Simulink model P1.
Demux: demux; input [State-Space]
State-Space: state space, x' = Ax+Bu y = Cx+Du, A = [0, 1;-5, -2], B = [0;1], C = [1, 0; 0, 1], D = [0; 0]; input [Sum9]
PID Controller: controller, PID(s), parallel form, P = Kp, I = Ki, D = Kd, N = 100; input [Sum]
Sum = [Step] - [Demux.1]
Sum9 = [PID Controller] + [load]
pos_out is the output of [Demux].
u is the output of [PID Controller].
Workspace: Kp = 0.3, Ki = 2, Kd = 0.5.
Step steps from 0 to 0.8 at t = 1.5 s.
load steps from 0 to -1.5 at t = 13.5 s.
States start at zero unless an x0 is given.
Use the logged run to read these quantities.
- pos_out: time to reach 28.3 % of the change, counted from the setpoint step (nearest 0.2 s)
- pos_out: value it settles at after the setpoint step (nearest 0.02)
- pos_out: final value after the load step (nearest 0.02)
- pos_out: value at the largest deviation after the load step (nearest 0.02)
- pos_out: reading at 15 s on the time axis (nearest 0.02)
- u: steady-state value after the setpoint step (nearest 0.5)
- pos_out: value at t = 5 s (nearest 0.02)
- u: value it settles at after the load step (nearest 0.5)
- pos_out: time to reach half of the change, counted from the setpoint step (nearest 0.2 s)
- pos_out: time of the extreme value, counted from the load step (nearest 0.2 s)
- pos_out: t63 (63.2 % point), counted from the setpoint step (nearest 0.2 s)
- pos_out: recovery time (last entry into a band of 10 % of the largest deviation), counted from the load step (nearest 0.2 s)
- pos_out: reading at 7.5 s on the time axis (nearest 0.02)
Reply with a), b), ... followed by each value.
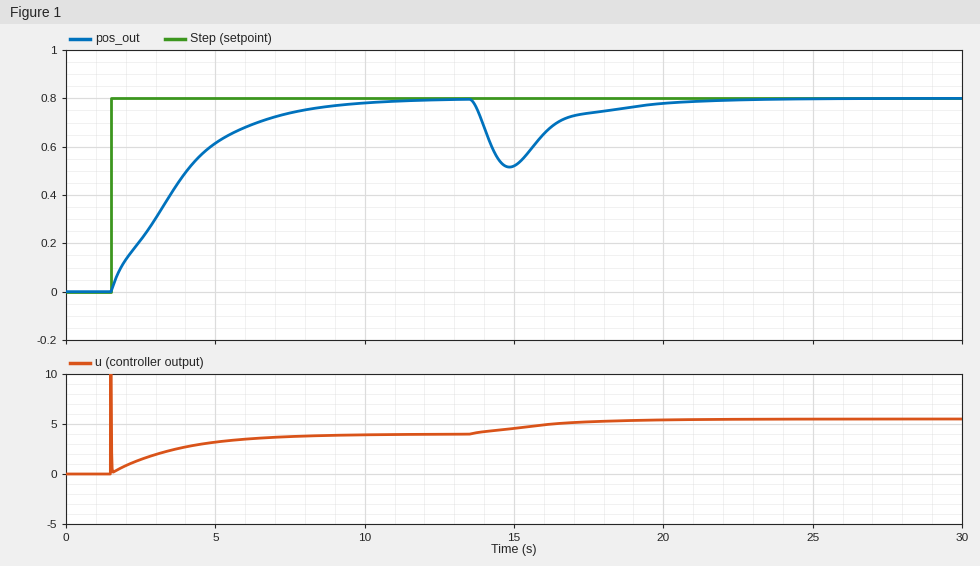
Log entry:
a) 1.0 s
b) 0.80
c) 0.80
d) 0.52
e) 0.52
f) 4.0
g) 0.62
h) 5.5
i) 2.0 s
j) 1.4 s
k) 2.6 s
l) 6.0 s
m) 0.74
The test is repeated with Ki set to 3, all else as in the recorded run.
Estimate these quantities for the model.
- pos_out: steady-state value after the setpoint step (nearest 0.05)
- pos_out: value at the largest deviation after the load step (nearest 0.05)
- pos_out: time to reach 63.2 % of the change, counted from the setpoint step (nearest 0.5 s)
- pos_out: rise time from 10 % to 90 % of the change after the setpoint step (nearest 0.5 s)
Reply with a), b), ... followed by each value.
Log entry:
a) 0.80
b) 0.55
c) 2.0 s
d) 3.0 s
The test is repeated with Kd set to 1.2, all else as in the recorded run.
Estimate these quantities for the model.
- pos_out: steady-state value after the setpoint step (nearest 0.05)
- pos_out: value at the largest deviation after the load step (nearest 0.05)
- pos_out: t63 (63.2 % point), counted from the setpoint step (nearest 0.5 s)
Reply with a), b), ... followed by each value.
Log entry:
a) 0.80
b) 0.55
c) 3.0 s
